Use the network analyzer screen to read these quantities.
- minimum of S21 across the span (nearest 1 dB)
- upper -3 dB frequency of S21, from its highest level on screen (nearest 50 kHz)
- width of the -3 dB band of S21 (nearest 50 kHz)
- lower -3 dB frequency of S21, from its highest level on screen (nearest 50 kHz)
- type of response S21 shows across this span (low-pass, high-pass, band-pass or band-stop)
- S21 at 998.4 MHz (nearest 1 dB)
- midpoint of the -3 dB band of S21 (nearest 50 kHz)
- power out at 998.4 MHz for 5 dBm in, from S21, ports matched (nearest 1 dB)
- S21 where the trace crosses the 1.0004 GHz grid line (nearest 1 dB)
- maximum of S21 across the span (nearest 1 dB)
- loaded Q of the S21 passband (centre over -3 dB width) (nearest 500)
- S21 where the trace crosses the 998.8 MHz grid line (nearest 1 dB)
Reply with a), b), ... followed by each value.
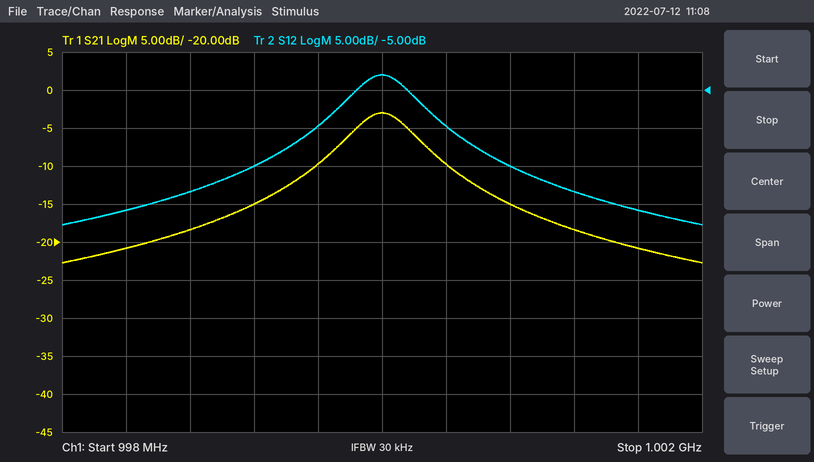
a) -23 dB
b) 1.00020 GHz
c) 400 kHz
d) 999.80 MHz
e) band-pass
f) -21 dB
g) 1.00000 GHz
h) -16 dBm
i) -10 dB
j) -3 dB
k) 2500
l) -18 dB
